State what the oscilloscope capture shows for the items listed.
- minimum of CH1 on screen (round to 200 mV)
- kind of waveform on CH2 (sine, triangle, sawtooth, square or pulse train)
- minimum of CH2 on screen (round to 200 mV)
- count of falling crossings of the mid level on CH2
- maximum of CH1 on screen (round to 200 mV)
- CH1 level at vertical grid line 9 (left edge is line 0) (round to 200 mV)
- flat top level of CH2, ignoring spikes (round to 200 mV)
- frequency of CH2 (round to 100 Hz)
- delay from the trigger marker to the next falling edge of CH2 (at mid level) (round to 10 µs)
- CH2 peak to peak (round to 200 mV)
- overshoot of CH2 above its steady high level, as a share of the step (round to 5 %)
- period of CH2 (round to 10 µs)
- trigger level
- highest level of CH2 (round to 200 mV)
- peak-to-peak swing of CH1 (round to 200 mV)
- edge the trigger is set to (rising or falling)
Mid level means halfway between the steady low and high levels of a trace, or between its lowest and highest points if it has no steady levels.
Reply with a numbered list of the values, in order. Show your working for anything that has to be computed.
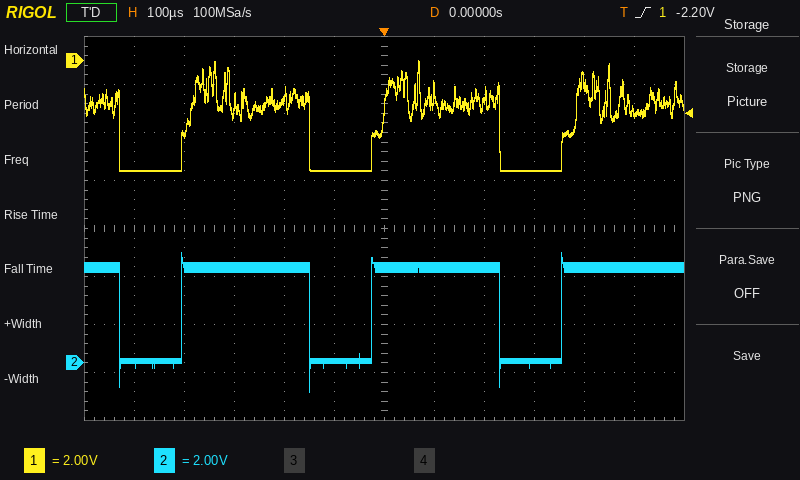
1. -4.6 V
2. pulse train
3. -1.2 V
4. 3
5. 0.0 V
6. -4.6 V
7. 4.0 V
8. 1 / 380 µs ≈ 2.6 kHz
9. 230 µs
10. 4.6 V − (-1.2 V) = 5.8 V
11. 15 %
12. 380 µs
13. -2.20 V
14. 4.6 V
15. 0.0 V − (-4.6 V) = 4.6 V
16. rising
